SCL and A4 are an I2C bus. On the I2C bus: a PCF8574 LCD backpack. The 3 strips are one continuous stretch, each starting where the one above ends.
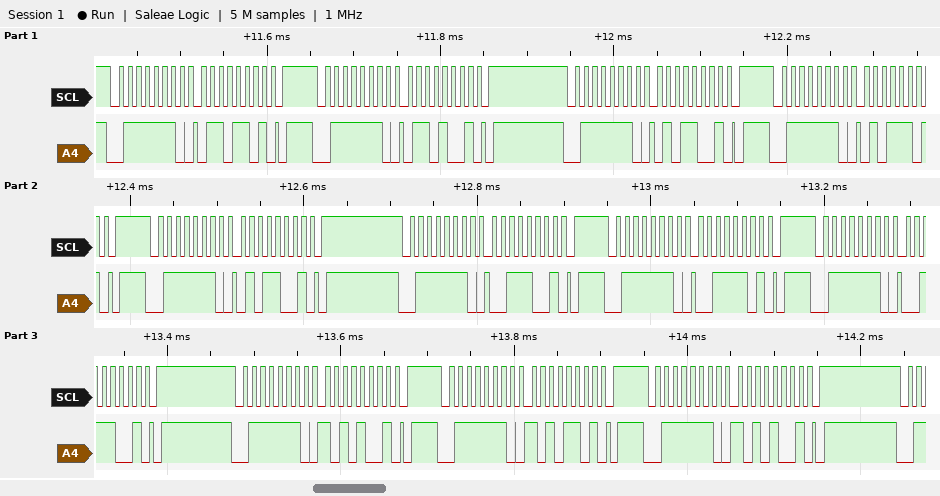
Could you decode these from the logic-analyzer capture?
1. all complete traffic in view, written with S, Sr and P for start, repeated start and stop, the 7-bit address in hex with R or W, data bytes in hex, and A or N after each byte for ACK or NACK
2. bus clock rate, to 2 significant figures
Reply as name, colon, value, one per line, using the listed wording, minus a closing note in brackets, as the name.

all complete traffic in view, written with S, Sr and P for start, repeated start and stop, the 7-bit address in hex with R or W, data bytes in hex, and A or N after each byte for ACK or NACK: S 3FW A 6D A P S 3FW A 69 A P S 3FW A 59 A P S 3FW A 5D A P S 3FW A 59 A P S 3FW A 39 A P S 3FW A 3D A P S 3FW A 39 A P S 3FW A A9 A P S 3FW A AD A P S 3FW A A9 A P
bus clock rate, to 2 significant figures: 100 kHz
